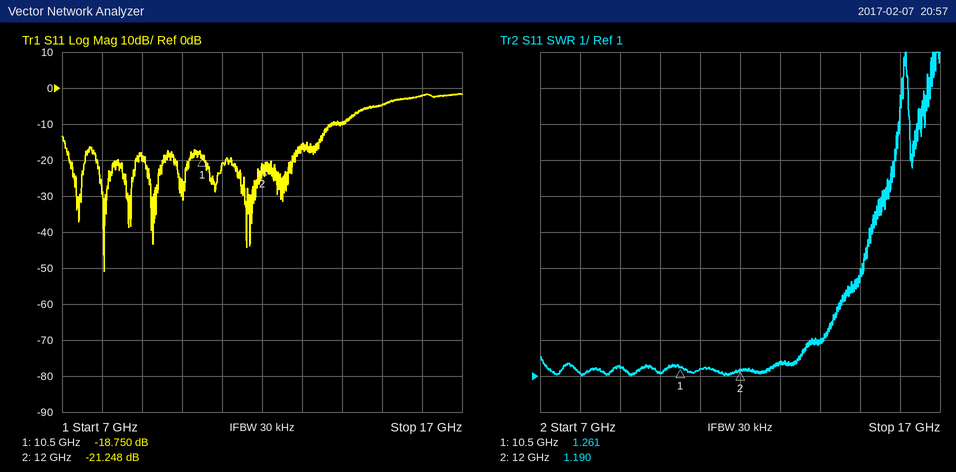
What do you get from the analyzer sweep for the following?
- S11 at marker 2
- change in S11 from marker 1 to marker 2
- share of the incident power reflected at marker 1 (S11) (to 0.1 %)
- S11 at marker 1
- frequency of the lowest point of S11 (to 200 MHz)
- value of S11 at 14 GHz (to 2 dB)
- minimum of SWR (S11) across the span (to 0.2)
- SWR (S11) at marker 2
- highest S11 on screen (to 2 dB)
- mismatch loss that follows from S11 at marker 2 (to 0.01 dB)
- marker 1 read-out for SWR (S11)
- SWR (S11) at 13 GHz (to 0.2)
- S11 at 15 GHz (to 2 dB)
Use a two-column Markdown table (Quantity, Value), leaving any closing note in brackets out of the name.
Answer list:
| Quantity | Value |
|---|---|
| S11 at marker 2 | -21.248 dB |
| change in S11 from marker 1 to marker 2 | -2.498 dB |
| share of the incident power reflected at marker 1 (S11) | 1.3 % |
| S11 at marker 1 | -18.750 dB |
| frequency of the lowest point of S11 | 8.0 GHz |
| value of S11 at 14 GHz | -10 dB |
| minimum of SWR (S11) across the span | 1.0 |
| SWR (S11) at marker 2 | 1.190 |
| highest S11 on screen | -2 dB |
| mismatch loss that follows from S11 at marker 2 | 0.03 dB |
| marker 1 read-out for SWR | 1.261 |
| SWR (S11) at 13 GHz | 1.4 |
| S11 at 15 GHz | -4 dB |
